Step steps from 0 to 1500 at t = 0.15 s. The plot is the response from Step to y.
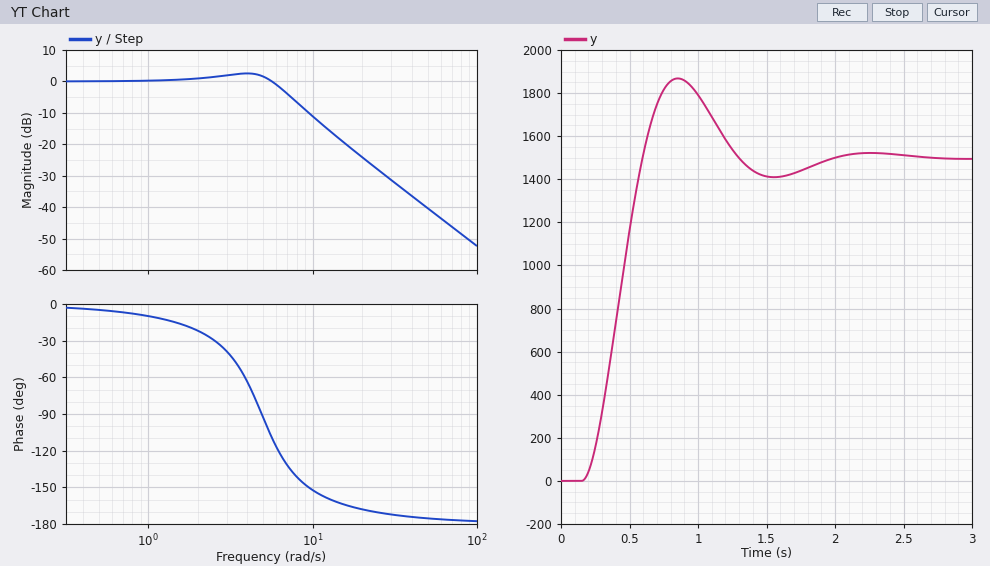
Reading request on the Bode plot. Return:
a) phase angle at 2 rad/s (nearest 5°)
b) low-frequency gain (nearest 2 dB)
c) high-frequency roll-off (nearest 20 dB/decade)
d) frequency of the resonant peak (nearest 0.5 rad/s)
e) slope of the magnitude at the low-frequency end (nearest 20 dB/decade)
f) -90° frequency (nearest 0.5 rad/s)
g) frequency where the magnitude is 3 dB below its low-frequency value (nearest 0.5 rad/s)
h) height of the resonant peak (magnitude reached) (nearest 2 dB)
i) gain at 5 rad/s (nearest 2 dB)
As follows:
-20°
0 dB
-40 dB/decade
4.0 rad/s
0 dB/decade
5.0 rad/s
6.5 rad/s
2 dB
2 dB
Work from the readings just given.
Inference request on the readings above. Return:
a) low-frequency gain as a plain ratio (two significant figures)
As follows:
1.0
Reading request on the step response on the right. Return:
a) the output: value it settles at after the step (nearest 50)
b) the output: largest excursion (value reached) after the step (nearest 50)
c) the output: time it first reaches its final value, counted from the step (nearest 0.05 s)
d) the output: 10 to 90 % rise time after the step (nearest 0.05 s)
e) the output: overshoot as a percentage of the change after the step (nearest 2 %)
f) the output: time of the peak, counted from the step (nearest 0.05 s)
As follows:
1500
1850
0.45 s
0.30 s
24 %
0.70 s
